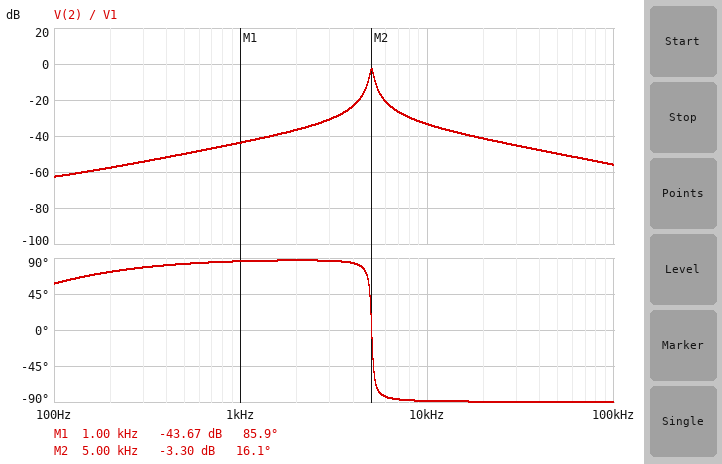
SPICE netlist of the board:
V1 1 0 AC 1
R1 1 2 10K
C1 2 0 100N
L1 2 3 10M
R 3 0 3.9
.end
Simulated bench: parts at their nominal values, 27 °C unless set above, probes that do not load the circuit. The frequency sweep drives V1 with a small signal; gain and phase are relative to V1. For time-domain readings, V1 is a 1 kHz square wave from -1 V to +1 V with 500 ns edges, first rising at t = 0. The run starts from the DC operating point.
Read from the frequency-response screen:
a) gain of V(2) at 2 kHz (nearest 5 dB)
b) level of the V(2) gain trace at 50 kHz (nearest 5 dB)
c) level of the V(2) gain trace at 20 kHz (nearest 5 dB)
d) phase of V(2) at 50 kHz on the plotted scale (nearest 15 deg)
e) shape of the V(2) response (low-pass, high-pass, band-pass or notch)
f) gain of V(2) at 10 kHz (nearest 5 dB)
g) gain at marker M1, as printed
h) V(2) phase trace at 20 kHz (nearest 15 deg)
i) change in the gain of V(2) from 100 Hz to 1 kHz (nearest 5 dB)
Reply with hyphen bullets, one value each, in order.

- -35 dB
- -50 dB
- -40 dB
- -90 deg
- band-pass
- -35 dB
- -43.67 dB
- -90 deg
- 20 dB
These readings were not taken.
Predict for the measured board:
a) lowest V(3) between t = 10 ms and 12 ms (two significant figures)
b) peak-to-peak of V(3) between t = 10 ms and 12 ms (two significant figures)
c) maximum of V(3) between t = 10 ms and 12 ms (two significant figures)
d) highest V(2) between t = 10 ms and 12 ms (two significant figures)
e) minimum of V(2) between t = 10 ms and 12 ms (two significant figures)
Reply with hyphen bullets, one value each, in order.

- -2.8 mV
- 5.6 mV
- 2.8 mV
- 200 mV
- -200 mV
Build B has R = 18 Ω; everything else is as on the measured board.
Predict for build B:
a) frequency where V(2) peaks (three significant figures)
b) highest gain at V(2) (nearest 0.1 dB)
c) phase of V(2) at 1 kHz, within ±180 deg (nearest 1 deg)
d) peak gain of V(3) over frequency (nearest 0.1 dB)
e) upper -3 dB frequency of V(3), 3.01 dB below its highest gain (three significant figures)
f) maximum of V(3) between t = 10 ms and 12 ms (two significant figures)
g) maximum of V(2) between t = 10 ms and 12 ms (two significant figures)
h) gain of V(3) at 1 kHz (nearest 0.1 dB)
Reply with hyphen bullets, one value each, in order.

- 5.04 kHz
- -8.9 dB
- 73 deg
- -33.8 dB
- 5.25 kHz
- 8.0 mV
- 120 mV
- -54.6 dB
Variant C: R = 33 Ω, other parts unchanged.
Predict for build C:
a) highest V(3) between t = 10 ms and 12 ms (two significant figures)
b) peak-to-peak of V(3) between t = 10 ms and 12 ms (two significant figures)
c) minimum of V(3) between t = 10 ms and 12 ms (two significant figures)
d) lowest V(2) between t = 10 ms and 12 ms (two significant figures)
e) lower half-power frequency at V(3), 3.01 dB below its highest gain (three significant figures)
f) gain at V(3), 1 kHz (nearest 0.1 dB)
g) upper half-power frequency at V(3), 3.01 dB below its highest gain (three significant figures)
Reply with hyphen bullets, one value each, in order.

- 11 mV
- 23 mV
- -11 mV
- -89 mV
- 4.66 kHz
- -49.3 dB
- 5.35 kHz
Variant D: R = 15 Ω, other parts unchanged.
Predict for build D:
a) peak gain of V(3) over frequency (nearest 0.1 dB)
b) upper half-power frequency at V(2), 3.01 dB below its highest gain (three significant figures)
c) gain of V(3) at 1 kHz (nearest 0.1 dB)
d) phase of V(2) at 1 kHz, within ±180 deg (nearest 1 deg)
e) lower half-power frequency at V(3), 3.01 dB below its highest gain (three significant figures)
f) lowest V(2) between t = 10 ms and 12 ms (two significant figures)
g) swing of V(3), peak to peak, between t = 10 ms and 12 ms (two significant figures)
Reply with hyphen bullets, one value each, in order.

- -34.4 dB
- 5.24 kHz
- -56.1 dB
- 76 deg
- 4.83 kHz
- -130 mV
- 14 mV
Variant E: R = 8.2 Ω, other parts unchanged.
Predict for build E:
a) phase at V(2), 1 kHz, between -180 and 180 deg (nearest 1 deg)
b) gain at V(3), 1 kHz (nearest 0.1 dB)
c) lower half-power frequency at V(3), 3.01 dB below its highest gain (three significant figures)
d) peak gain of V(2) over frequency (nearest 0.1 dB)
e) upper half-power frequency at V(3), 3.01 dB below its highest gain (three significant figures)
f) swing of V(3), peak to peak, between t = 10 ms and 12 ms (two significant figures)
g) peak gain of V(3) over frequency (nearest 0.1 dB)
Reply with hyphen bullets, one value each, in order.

- 82 deg
- -61.4 dB
- 4.88 kHz
- -5.2 dB
- 5.17 kHz
- 9.7 mV
- -36.9 dB
